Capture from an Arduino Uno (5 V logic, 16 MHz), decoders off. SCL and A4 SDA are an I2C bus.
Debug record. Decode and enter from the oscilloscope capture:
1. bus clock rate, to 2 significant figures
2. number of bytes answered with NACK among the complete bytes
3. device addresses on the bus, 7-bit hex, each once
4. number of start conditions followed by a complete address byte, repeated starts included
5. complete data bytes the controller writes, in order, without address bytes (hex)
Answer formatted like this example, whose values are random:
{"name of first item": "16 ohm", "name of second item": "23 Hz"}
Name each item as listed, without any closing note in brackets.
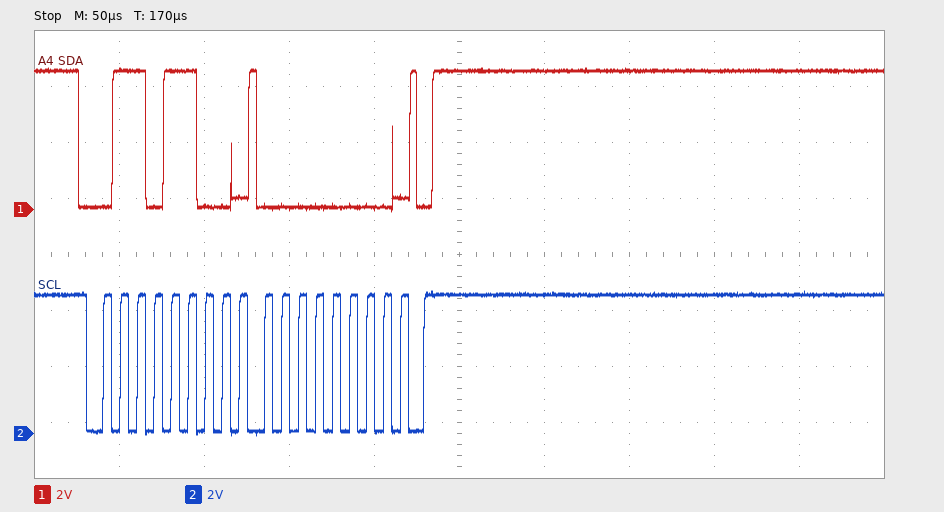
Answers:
{"bus clock rate, to 2 significant figures": "100 kHz", "number of bytes answered with NACK among the complete bytes": "0", "device addresses on the bus, 7-bit hex, each once": "0x36", "number of start conditions followed by a complete address byte, repeated starts included": "1", "complete data bytes the controller writes, in order, without address bytes": "00"}
